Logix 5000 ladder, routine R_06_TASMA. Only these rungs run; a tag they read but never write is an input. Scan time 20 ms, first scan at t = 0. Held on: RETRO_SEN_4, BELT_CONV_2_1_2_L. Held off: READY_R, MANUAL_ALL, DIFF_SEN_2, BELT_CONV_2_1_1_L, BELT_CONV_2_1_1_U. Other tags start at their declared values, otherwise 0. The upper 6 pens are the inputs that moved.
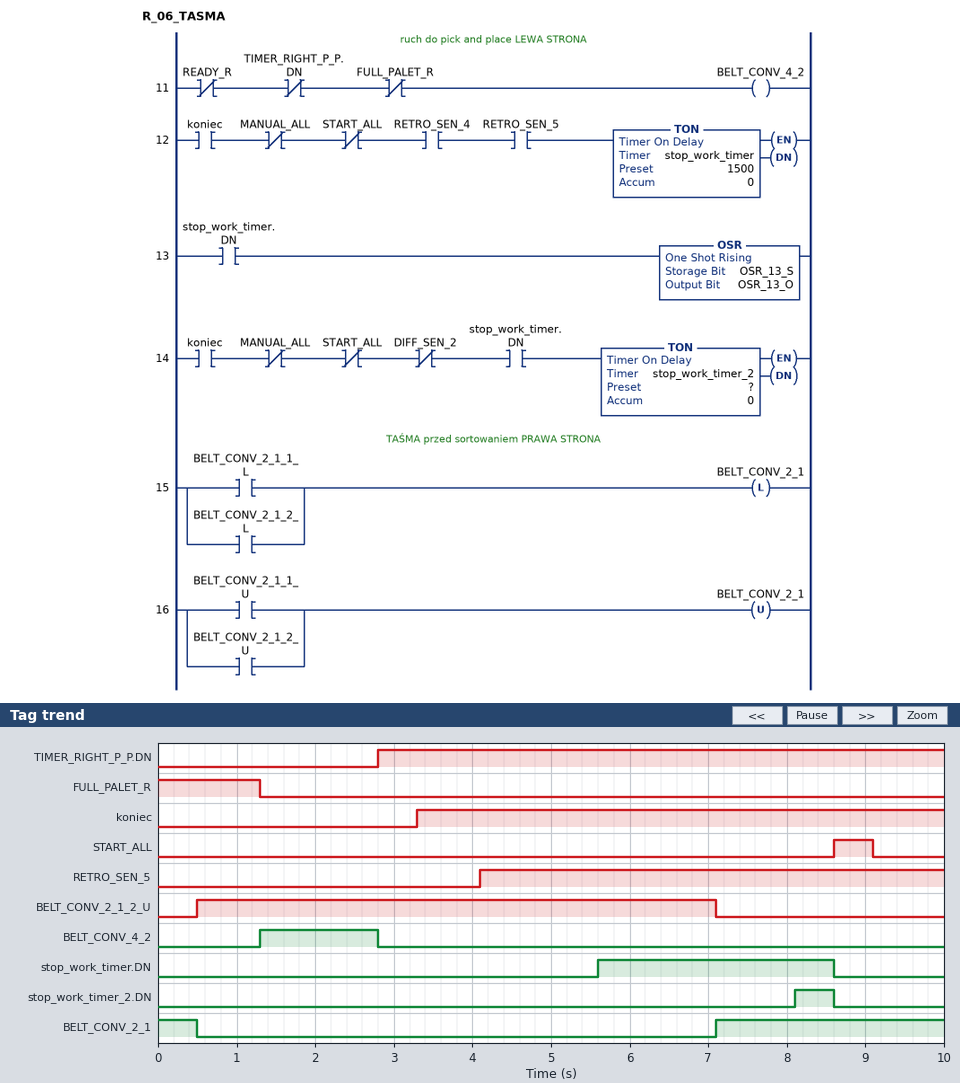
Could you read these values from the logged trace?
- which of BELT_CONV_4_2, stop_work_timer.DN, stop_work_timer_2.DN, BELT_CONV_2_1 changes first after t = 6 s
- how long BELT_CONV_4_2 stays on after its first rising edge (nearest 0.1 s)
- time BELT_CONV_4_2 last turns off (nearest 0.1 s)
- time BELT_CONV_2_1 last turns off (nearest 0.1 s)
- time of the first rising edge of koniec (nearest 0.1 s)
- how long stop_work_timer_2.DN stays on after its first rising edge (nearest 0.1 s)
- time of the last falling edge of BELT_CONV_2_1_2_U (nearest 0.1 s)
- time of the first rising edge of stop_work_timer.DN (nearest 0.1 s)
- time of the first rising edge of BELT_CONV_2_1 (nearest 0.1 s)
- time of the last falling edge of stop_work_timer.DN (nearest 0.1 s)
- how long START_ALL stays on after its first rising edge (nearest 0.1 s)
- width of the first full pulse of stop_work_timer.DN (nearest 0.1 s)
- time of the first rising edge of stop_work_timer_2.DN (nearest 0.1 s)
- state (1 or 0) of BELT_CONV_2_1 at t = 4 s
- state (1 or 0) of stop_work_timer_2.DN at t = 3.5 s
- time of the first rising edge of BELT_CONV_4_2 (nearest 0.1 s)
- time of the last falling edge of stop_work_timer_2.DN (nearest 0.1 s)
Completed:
BELT_CONV_2_1
1.5 s
2.8 s
0.5 s
3.3 s
0.5 s
7.1 s
5.6 s
7.1 s
8.6 s
0.5 s
3.0 s
8.1 s
0
0
1.3 s
8.6 s
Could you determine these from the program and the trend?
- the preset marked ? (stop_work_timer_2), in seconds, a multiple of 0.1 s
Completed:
2.5 s
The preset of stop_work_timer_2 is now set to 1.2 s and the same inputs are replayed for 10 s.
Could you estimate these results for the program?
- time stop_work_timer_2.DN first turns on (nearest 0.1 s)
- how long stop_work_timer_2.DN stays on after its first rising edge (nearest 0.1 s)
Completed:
6.8 s
1.8 s
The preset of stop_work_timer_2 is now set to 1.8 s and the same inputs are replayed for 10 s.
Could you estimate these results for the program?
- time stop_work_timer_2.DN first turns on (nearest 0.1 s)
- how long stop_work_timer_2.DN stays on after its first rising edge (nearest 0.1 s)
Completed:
7.4 s
1.2 s
